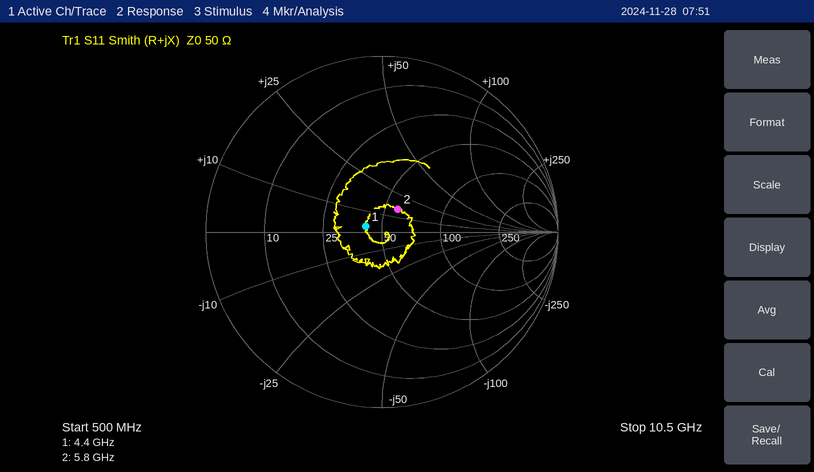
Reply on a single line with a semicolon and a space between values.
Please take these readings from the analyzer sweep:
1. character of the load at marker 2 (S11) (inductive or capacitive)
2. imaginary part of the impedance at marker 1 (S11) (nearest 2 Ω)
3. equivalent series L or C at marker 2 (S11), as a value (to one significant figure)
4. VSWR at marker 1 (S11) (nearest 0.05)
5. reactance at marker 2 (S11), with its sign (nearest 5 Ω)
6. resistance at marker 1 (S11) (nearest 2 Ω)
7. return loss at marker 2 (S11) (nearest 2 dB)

inductive; +2 Ω; 400 pH; 1.20; +15 Ω; 42 Ω; 16 dB
